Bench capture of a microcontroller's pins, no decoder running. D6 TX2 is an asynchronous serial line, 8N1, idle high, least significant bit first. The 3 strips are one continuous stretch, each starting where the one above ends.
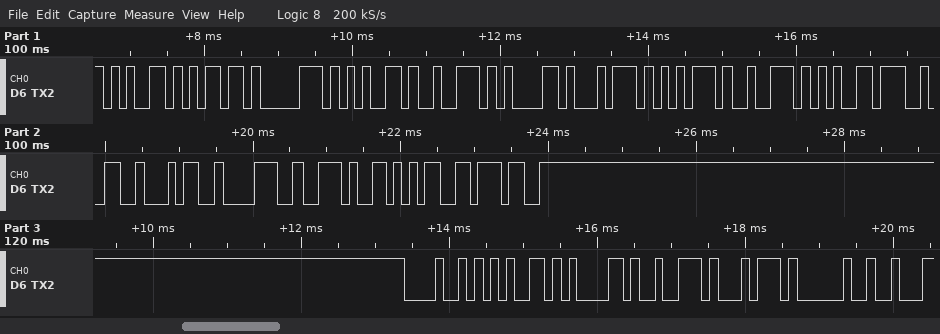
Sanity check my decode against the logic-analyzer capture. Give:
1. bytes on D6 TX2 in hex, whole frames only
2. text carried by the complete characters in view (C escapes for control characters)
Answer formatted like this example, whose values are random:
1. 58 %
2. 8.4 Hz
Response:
1. 0x65 0x6D 0x70 0x65 0x72 0x61 0x74 0x75 0x72 0x65 0x32 0x34 0x38 0x2E 0x35 0x37 0x48 0x65 0x61 0x72 0x74 0x20
2. "emperature248.57Heart "
